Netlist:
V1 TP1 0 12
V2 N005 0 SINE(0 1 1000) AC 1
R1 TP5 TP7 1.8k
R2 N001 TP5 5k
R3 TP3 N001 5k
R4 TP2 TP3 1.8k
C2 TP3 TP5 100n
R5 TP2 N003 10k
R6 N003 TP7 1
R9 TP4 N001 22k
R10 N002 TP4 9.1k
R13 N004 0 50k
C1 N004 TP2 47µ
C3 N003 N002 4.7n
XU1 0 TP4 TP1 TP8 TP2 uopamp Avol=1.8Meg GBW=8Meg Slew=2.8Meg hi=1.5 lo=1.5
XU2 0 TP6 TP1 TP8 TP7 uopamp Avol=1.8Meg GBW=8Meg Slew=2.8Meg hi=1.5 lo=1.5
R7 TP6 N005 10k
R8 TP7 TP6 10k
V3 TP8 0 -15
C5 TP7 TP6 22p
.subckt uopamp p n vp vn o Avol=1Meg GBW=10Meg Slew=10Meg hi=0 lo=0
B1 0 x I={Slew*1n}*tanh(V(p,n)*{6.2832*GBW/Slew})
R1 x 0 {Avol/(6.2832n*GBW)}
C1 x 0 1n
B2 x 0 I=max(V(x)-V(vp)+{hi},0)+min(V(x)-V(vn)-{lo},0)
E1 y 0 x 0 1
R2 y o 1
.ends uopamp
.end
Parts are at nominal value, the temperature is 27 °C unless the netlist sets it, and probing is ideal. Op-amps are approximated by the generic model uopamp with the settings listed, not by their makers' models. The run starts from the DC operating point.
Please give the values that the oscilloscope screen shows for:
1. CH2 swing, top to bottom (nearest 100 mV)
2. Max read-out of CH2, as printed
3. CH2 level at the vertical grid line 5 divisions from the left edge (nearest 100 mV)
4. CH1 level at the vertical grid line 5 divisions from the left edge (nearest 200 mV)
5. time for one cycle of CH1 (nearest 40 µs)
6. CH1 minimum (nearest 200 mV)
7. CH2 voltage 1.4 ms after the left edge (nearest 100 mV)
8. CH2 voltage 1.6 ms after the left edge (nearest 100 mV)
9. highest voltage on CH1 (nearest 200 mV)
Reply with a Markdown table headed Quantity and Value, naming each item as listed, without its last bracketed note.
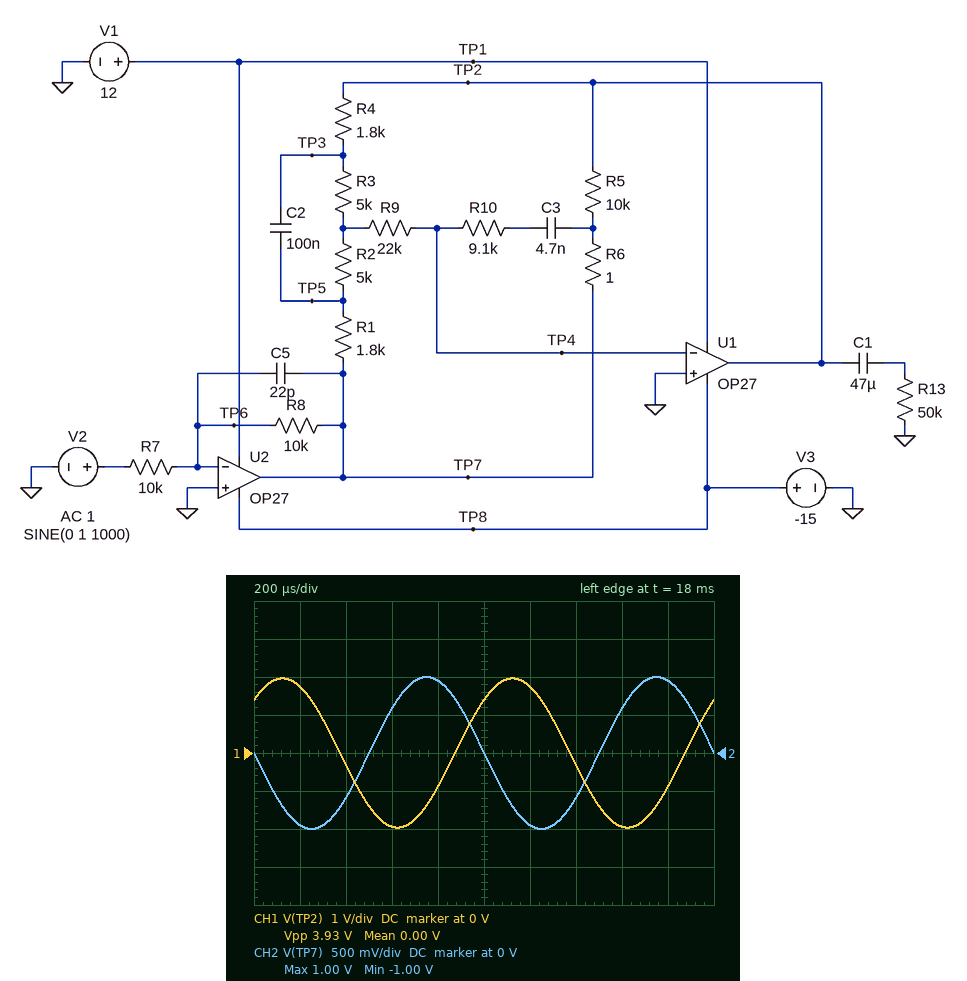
| Quantity | Value |
|---|---|
| CH2 swing, top to bottom | 2.0 V |
| Max read-out of CH2, as printed | 1.00 V |
| CH2 level at the vertical grid line 5 divisions from the left edge | 0 V |
| CH1 level at the vertical grid line 5 divisions from the left edge | 1.4 V |
| time for one cycle of CH1 | 1.00 ms |
| CH1 minimum | -2.0 V |
| CH2 voltage 1.4 ms after the left edge | -600 mV |
| CH2 voltage 1.6 ms after the left edge | 600 mV |
| highest voltage on CH1 | 2.0 V |
